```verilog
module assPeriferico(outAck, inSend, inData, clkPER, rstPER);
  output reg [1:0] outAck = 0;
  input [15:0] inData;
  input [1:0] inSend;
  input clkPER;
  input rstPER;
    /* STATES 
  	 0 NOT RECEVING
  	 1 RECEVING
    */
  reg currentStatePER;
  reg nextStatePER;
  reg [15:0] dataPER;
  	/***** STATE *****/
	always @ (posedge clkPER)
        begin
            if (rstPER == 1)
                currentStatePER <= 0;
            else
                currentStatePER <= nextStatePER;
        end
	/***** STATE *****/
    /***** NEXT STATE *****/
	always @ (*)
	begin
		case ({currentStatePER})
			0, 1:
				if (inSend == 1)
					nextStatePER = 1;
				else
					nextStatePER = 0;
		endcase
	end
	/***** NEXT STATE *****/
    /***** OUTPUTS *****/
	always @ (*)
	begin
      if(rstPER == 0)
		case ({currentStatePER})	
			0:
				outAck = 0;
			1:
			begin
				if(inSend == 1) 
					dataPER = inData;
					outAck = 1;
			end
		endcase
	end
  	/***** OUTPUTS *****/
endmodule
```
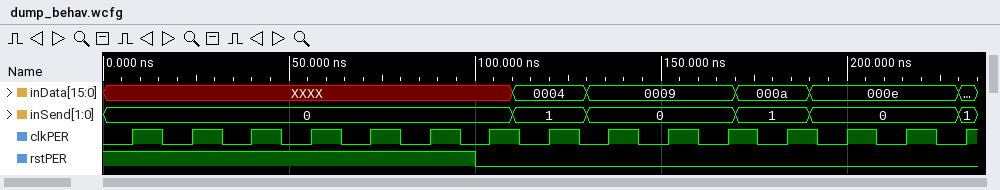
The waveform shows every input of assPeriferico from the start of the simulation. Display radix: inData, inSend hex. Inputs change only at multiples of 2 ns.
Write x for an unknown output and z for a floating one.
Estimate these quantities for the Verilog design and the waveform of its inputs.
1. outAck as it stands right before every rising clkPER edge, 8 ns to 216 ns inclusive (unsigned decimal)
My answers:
0, 0, 0, 0, 0, 0, 0, 0, 1, 0, 0, 0, 1, 0
